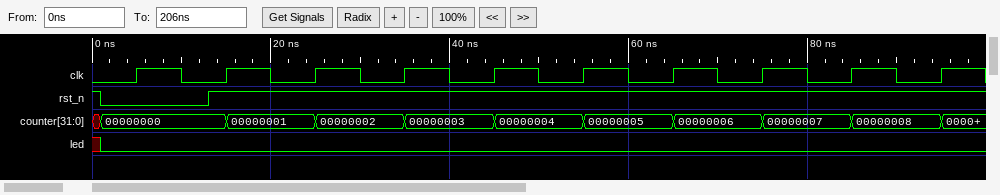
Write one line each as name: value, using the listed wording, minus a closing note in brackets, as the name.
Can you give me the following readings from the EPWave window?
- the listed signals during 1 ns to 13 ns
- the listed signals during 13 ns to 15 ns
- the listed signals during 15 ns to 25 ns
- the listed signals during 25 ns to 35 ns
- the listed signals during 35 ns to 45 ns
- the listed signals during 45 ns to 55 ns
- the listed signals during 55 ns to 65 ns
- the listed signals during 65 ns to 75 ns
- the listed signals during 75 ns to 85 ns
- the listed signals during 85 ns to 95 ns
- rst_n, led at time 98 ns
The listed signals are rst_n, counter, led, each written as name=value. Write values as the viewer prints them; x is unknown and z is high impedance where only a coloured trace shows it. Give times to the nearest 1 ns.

the listed signals during 1 ns to 13 ns: rst_n=0, counter=00000000, led=0
the listed signals during 13 ns to 15 ns: rst_n=1, counter=00000000, led=0
the listed signals during 15 ns to 25 ns: rst_n=1, counter=00000001, led=0
the listed signals during 25 ns to 35 ns: rst_n=1, counter=00000002, led=0
the listed signals during 35 ns to 45 ns: rst_n=1, counter=00000003, led=0
the listed signals during 45 ns to 55 ns: rst_n=1, counter=00000004, led=0
the listed signals during 55 ns to 65 ns: rst_n=1, counter=00000005, led=0
the listed signals during 65 ns to 75 ns: rst_n=1, counter=00000006, led=0
the listed signals during 75 ns to 85 ns: rst_n=1, counter=00000007, led=0
the listed signals during 85 ns to 95 ns: rst_n=1, counter=00000008, led=0
rst_n, led at time 98 ns: rst_n=1, led=0
